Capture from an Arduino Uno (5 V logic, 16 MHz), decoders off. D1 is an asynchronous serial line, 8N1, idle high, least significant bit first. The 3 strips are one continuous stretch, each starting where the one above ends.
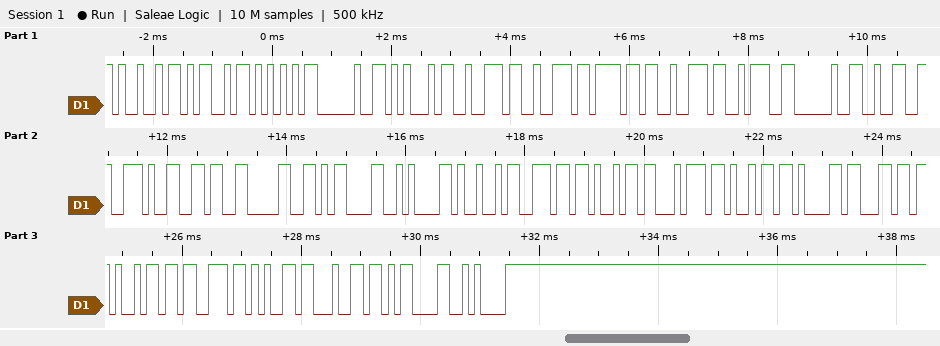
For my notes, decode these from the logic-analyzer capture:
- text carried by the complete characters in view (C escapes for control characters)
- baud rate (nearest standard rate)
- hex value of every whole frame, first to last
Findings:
"IMU Error: 2.60\r\nInitialised\r\n"
9600 baud
49 4D 55 20 45 72 72 6F 72 3A 20 32 2E 36 30 0D 0A 49 6E 69 74 69 61 6C 69 73 65 64 0D 0A
